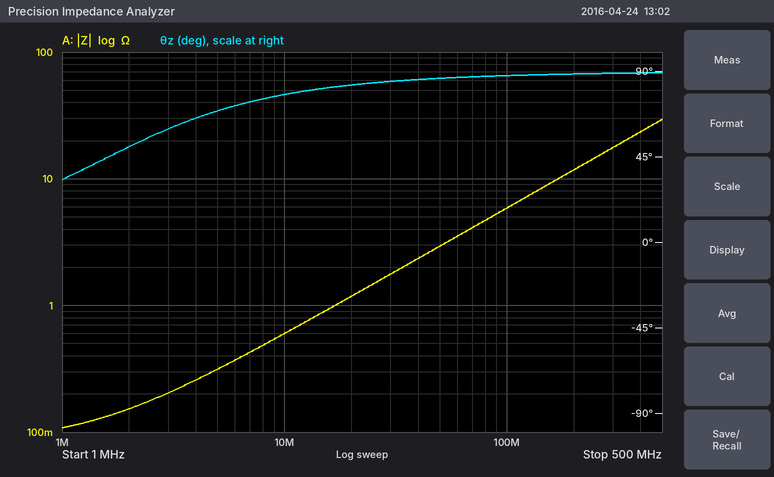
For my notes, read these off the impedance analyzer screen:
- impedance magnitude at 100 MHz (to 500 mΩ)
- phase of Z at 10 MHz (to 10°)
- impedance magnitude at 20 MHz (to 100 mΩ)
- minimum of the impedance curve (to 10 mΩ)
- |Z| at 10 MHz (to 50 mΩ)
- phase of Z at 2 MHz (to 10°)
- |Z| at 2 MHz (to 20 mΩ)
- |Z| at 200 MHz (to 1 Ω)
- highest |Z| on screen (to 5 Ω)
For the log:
6.0 Ω
80°
1.2 Ω
110 mΩ
600 mΩ
50°
160 mΩ
12 Ω
30 Ω
